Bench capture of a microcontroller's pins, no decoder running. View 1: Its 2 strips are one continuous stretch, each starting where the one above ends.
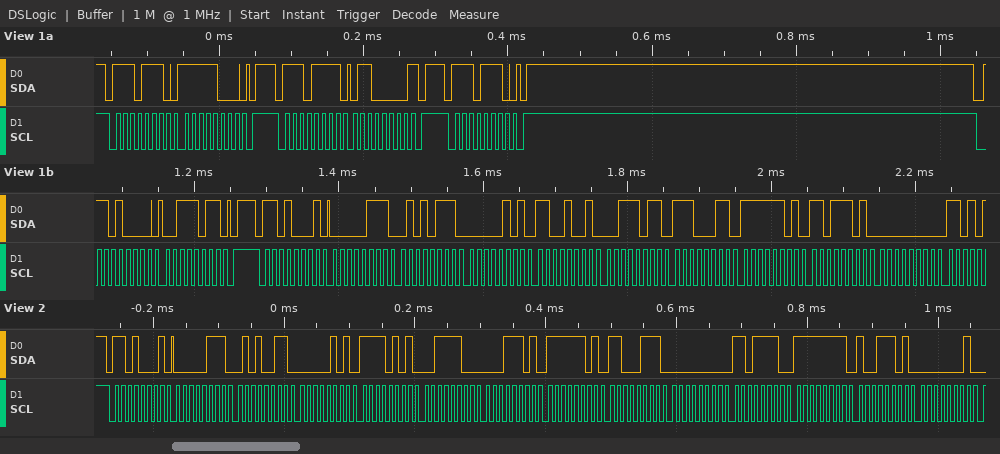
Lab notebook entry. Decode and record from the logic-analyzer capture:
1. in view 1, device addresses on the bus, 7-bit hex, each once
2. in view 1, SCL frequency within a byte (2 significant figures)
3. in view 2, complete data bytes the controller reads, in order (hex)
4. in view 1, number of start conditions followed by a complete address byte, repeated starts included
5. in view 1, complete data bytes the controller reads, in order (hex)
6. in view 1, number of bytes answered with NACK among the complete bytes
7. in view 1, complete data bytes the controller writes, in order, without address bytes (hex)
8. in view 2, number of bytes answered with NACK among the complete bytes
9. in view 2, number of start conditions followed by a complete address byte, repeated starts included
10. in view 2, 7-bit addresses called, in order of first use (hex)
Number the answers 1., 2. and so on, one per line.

1. 0x77 0x68
2. 100 kHz
3. 07 53 05 F5 3C 1D FD C7 00 DE FF 9D 01
4. 5
5. 60 07 57 05 C9 3B E3 FD DD 00
6. 1
7. F8 3B
8. 0
9. 1
10. 0x68
